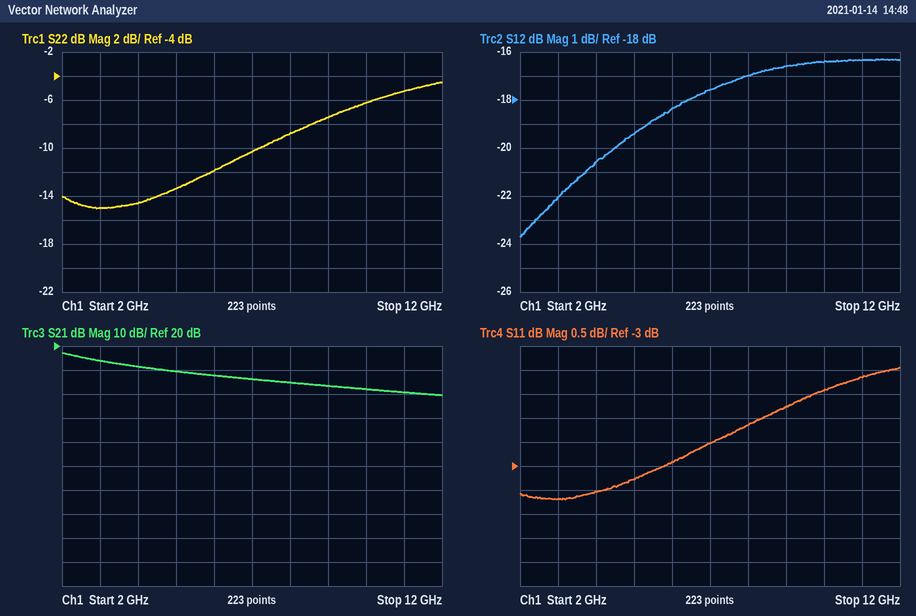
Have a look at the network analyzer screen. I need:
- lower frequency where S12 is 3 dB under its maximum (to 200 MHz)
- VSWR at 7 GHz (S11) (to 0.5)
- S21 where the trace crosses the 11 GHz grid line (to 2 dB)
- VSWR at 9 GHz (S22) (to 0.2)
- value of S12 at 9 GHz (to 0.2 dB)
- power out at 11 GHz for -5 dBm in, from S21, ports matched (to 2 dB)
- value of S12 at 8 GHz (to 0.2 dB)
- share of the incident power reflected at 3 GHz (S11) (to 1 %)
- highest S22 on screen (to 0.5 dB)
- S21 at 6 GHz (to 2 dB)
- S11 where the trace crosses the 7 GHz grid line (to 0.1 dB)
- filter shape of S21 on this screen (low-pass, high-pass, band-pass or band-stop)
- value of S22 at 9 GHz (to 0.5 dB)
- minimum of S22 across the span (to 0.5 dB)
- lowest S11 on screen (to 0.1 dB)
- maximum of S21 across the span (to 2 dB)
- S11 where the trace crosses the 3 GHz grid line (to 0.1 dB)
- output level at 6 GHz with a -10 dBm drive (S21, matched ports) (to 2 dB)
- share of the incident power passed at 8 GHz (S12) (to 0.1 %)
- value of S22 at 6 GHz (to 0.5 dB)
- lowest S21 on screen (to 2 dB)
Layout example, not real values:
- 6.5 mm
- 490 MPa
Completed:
- 5.0 GHz
- 7.0
- 0 dB
- 2.4
- -16.6 dB
- -4 dBm
- -17.0 dB
- 43 %
- -4.5 dB
- 8 dB
- -2.5 dB
- low-pass
- -7.5 dB
- -15.0 dB
- -3.7 dB
- 18 dB
- -3.7 dB
- -2 dBm
- 2.0 %
- -12.0 dB
- 0 dB
